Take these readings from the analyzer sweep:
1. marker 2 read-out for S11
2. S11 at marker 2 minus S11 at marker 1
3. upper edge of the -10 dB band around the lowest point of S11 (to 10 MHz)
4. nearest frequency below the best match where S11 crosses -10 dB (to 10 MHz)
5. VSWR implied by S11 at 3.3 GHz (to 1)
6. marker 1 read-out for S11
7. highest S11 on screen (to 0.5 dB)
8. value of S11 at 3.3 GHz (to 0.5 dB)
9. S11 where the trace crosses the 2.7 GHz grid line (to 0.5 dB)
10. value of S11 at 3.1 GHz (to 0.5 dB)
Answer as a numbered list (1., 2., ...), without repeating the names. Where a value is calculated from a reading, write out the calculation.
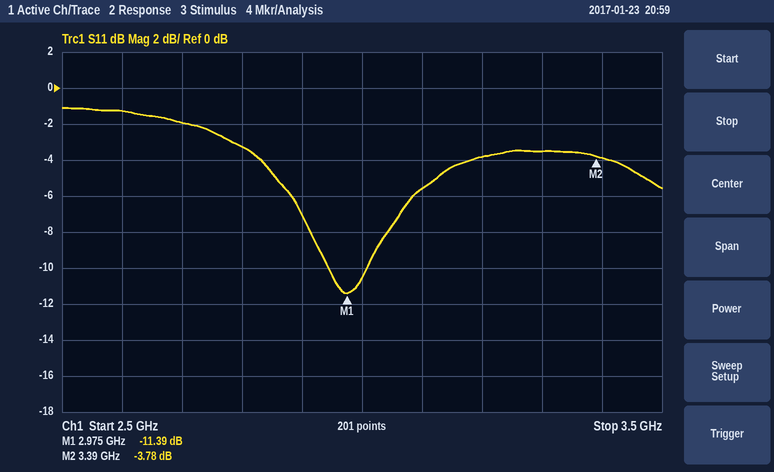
1. -3.78 dB
2. -3.78 − (-11.39) = 7.61 dB
3. 3.01 GHz
4. 2.94 GHz
5. |Γ| = 10^(-3.5/20) = 0.6683; VSWR = (1 + 0.6683)/(1 − 0.6683) ≈ 5
6. -11.39 dB
7. -1.0 dB
8. -3.5 dB
9. -2.0 dB
10. -5.5 dB
